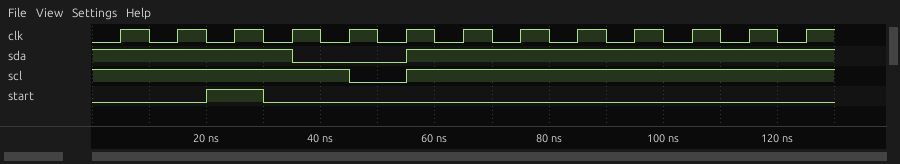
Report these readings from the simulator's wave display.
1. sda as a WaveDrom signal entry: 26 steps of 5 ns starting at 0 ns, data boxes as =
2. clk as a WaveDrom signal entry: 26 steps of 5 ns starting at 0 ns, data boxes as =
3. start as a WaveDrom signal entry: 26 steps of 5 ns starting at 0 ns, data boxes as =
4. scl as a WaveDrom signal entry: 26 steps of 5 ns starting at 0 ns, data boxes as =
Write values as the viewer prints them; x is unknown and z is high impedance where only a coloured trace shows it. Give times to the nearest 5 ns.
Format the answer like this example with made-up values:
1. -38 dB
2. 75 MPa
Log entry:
1. {name: 'sda', wave: '1......0...1..............'}
2. {name: 'clk', wave: '01010101010101010101010101'}
3. {name: 'start', wave: '0...1.0...................'}
4. {name: 'scl', wave: '1........0.1..............'}
